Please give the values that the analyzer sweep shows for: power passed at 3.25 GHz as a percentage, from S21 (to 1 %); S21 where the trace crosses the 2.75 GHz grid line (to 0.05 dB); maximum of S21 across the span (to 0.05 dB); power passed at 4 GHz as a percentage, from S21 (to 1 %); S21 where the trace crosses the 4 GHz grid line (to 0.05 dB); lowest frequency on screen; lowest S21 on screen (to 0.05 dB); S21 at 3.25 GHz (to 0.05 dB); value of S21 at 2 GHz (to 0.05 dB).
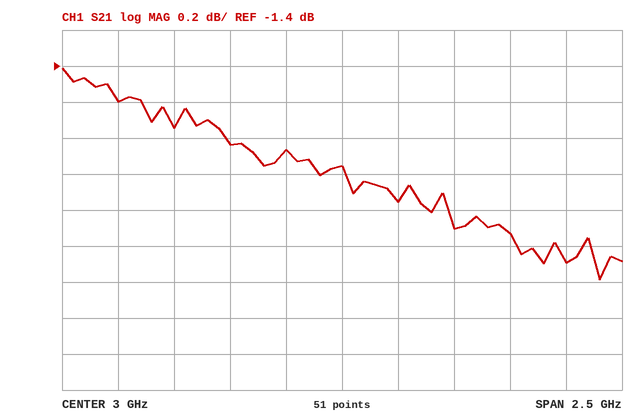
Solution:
61 %
-1.85 dB
-1.40 dB
56 %
-2.50 dB
1.75 GHz
-2.60 dB
-2.15 dB
-1.60 dB
